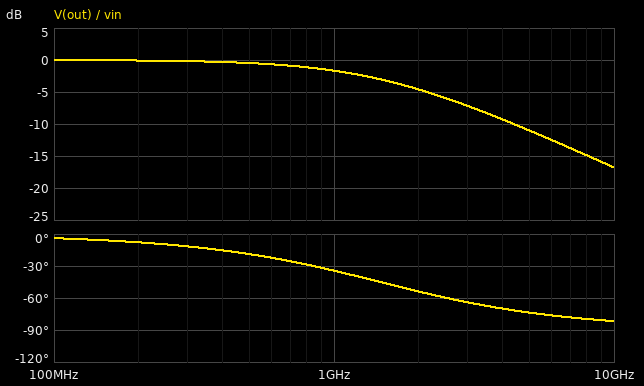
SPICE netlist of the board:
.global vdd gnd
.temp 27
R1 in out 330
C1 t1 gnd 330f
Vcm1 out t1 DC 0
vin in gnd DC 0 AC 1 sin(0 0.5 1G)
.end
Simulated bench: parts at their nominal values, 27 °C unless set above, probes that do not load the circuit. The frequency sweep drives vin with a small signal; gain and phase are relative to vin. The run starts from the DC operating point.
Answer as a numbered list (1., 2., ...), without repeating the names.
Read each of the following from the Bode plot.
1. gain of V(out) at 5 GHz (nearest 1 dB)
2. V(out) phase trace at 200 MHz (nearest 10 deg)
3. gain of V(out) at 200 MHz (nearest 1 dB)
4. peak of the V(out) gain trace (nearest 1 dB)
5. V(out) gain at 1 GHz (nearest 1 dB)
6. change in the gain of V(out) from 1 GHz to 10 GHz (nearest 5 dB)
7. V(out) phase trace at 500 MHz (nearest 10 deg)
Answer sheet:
1. -11 dB
2. -10 deg
3. 0 dB
4. 0 dB
5. -2 dB
6. -15 dB
7. -20 deg
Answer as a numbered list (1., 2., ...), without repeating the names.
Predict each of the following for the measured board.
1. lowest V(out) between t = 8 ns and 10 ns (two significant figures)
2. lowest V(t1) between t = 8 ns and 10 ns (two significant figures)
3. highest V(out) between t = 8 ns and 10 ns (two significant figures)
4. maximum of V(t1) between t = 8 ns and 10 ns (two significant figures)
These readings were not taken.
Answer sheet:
1. -410 mV
2. -410 mV
3. 410 mV
4. 410 mV
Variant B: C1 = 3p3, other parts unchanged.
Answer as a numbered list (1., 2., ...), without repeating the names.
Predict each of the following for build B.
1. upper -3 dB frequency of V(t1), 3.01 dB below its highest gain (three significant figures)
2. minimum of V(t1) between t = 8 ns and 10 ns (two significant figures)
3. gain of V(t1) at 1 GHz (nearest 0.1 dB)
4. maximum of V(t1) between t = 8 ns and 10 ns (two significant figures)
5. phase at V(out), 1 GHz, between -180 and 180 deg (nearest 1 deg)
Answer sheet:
1. 146 MHz
2. -72 mV
3. -16.8 dB
4. 72 mV
5. -82 deg
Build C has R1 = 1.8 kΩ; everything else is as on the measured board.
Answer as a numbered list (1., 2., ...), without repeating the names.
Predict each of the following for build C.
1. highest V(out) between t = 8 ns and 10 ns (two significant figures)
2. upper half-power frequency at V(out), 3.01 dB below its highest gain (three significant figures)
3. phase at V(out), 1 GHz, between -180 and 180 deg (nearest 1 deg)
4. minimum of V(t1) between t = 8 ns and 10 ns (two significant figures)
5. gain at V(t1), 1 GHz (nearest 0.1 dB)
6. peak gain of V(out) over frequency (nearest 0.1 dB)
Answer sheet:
1. 130 mV
2. 268 MHz
3. -75 deg
4. -130 mV
5. -11.7 dB
6. 0 dB
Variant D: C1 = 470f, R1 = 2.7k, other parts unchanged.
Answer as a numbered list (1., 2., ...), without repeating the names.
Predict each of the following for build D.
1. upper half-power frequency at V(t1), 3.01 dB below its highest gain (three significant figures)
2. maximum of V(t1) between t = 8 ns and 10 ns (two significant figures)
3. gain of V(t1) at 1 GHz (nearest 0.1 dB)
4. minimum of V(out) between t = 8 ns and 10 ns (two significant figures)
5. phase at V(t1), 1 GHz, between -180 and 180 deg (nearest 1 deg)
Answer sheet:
1. 125 MHz
2. 62 mV
3. -18.1 dB
4. -62 mV
5. -83 deg
